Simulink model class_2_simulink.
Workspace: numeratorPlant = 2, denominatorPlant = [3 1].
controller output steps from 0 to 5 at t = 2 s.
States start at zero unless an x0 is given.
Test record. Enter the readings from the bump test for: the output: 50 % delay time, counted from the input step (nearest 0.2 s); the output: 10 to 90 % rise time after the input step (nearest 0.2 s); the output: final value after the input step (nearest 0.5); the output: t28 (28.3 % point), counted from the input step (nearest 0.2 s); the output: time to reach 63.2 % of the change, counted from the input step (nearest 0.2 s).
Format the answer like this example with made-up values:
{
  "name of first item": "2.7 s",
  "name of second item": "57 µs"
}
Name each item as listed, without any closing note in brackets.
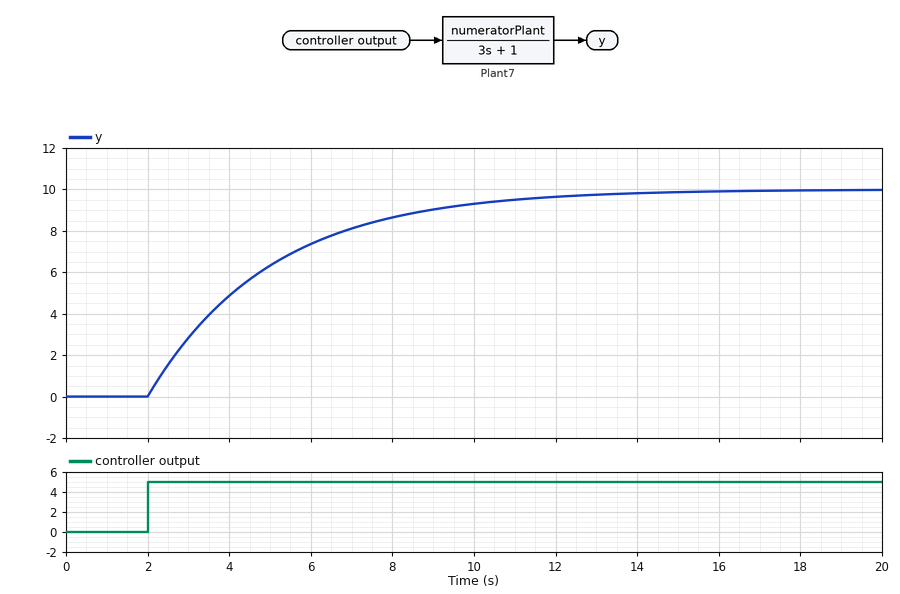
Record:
{
  "the output: 50 % delay time, counted from the input step": "2.0 s",
  "the output: 10 to 90 % rise time after the input step": "6.6 s",
  "the output: final value after the input step": "10.0",
  "the output: t28 (28.3 % point), counted from the input step": "1.0 s",
  "the output: time to reach 63.2 % of the change, counted from the input step": "3.0 s"
}
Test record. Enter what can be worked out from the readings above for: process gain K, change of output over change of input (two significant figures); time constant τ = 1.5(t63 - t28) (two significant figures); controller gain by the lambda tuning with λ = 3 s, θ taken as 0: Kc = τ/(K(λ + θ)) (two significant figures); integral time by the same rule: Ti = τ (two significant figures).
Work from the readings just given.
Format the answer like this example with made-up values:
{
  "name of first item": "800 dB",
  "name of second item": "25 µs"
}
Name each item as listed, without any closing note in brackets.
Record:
{
  "process gain K, change of output over change of input": "2.0",
  "time constant τ = 1.5(t63 - t28)": "3.0 s",
  "controller gain by the lambda tuning with λ = 3 s, θ taken as 0: Kc = τ/(K(λ + θ))": "0.50",
  "integral time by the same rule: Ti = τ": "3.0 s"
}
